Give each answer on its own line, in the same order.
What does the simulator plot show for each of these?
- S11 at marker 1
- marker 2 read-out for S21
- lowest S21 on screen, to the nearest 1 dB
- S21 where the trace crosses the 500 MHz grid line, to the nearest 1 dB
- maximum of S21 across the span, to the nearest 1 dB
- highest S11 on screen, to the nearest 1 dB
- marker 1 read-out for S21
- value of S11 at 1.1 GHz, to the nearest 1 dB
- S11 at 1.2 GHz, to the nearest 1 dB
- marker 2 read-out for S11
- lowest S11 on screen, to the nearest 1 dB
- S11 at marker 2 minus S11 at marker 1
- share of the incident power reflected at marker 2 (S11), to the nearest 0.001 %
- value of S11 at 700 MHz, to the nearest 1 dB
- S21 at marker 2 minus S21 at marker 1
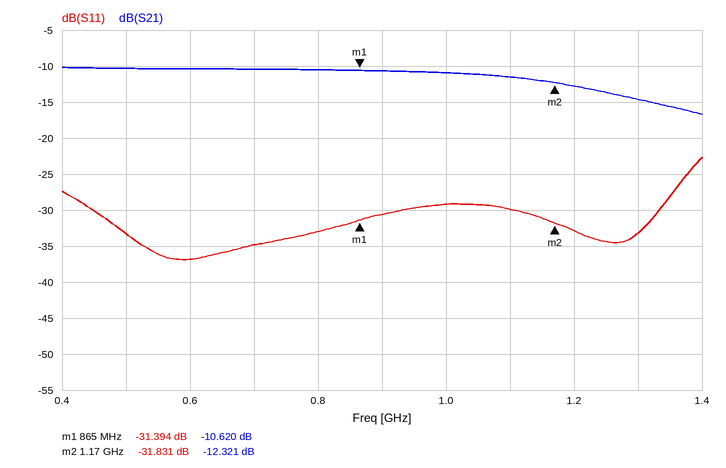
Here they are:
-31.394 dB
-12.321 dB
-17 dB
-10 dB
-10 dB
-23 dB
-10.620 dB
-30 dB
-33 dB
-31.831 dB
-37 dB
-0.437 dB
0.066 %
-35 dB
-1.701 dB
